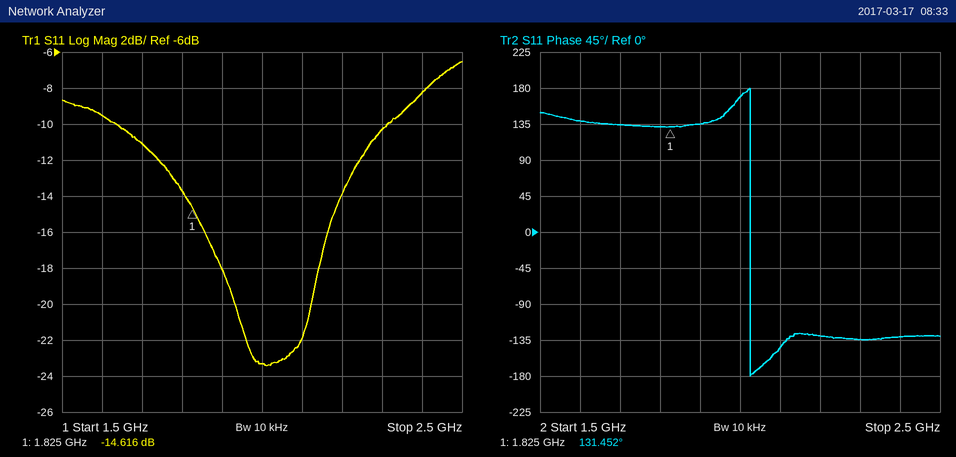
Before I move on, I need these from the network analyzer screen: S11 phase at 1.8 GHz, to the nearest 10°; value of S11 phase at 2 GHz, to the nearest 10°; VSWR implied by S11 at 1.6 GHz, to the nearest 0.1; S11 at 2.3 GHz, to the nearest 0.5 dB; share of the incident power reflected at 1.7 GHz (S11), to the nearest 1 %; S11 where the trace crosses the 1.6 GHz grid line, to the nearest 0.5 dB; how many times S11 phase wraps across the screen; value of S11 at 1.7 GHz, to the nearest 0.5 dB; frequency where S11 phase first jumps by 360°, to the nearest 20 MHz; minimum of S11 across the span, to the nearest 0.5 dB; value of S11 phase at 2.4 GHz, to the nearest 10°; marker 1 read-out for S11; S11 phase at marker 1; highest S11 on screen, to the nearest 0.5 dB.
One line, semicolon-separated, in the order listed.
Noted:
130°; 170°; 2.0; -10.5 dB; 8 %; -9.5 dB; 1; -11.0 dB; 2.02 GHz; -23.5 dB; -130°; -14.616 dB; 131.452°; -6.5 dB
